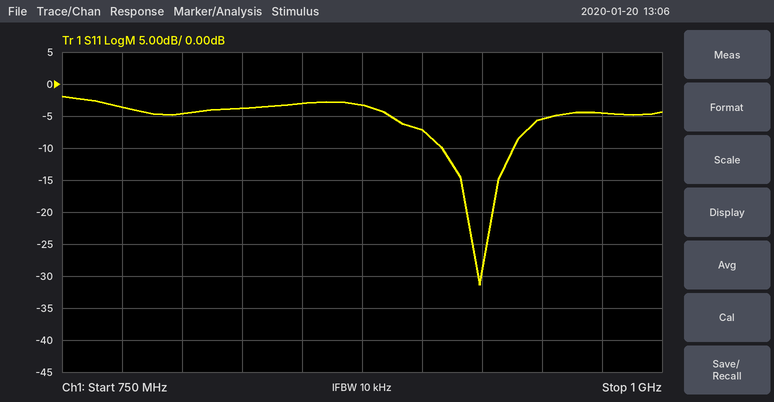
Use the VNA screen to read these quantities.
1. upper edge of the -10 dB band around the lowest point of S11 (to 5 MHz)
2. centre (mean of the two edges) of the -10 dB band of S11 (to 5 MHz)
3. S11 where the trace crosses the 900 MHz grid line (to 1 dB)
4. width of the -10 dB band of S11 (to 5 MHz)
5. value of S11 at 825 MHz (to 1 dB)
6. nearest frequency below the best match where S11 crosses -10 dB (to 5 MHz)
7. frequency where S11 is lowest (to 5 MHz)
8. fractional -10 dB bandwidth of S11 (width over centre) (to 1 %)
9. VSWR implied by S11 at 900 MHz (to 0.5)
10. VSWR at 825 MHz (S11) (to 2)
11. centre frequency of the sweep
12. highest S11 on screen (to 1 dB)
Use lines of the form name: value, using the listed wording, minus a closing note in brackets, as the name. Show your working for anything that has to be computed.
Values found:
upper edge of the -10 dB band around the lowest point of S11: 940 MHz
centre (mean of the two edges) of the -10 dB band of S11: 925 MHz
S11 where the trace crosses the 900 MHz grid line: -7 dB
width of the -10 dB band of S11: 940 MHz − 910 MHz = 30 MHz
value of S11 at 825 MHz: -4 dB
nearest frequency below the best match where S11 crosses -10 dB: 910 MHz
frequency where S11 is lowest: 925 MHz
fractional -10 dB bandwidth of S11 (width over centre): 30 MHz / 925 MHz ≈ 3 %
VSWR implied by S11 at 900 MHz: |Γ| = 10^(-7/20) = 0.4467; VSWR = (1 + 0.4467)/(1 − 0.4467) ≈ 2.61, so 2.5 to the nearest 0.5
VSWR at 825 MHz (S11): |Γ| = 10^(-4/20) = 0.6310; VSWR = (1 + 0.6310)/(1 − 0.6310) ≈ 4
centre frequency of the sweep: 875 MHz
highest S11 on screen: -2 dB
